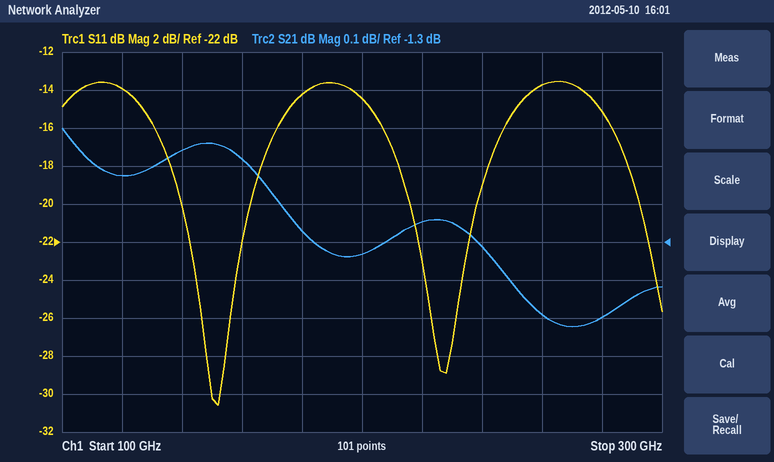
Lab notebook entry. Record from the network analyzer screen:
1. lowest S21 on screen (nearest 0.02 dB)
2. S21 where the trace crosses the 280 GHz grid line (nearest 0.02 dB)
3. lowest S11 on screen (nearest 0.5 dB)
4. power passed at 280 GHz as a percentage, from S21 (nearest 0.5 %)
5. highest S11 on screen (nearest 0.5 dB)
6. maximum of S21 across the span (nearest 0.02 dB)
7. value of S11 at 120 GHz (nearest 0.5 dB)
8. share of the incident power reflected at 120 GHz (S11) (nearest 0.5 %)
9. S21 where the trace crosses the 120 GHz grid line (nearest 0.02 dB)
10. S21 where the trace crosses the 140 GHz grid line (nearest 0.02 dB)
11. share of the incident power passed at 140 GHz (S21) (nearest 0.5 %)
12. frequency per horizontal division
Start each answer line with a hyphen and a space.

- -1.52 dB
- -1.50 dB
- -30.5 dB
- 71.0 %
- -13.5 dB
- -1.00 dB
- -14.0 dB
- 4.0 %
- -1.12 dB
- -1.06 dB
- 78.5 %
- 20 GHz
